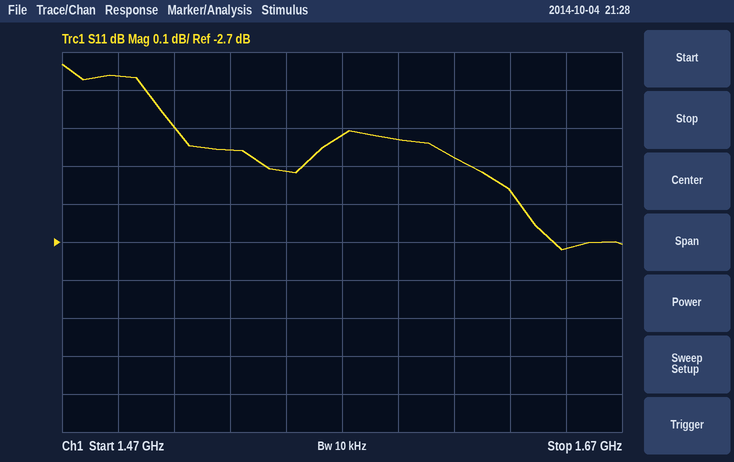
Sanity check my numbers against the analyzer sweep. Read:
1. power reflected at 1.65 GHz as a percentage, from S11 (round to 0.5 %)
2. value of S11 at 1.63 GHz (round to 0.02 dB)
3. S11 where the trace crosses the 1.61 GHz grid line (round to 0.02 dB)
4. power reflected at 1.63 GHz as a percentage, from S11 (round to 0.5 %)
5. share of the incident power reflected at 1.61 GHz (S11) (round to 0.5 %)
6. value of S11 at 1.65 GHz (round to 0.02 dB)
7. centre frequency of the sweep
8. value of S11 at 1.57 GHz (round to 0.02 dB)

53.5 %
-2.56 dB
-2.48 dB
55.5 %
56.5 %
-2.72 dB
1.57 GHz
-2.42 dB
